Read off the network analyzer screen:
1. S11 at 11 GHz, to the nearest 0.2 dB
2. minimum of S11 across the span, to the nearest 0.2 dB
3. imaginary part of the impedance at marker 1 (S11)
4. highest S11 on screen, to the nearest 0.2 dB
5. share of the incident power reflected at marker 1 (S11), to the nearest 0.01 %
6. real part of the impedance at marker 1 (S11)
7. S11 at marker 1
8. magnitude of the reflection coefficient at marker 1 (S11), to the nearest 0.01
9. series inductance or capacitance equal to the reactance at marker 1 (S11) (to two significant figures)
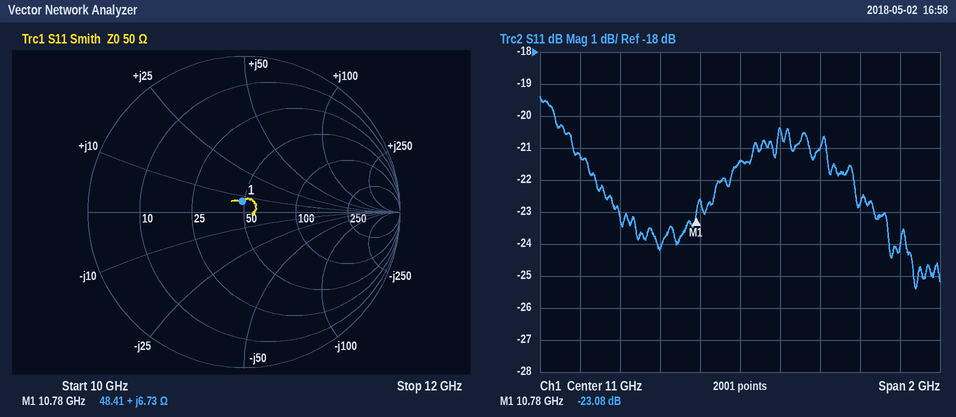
-21.4 dB
-25.4 dB
+6.73 Ω
-19.4 dB
0.49 %
48.41 Ω
-23.08 dB
0.07
99 pH
